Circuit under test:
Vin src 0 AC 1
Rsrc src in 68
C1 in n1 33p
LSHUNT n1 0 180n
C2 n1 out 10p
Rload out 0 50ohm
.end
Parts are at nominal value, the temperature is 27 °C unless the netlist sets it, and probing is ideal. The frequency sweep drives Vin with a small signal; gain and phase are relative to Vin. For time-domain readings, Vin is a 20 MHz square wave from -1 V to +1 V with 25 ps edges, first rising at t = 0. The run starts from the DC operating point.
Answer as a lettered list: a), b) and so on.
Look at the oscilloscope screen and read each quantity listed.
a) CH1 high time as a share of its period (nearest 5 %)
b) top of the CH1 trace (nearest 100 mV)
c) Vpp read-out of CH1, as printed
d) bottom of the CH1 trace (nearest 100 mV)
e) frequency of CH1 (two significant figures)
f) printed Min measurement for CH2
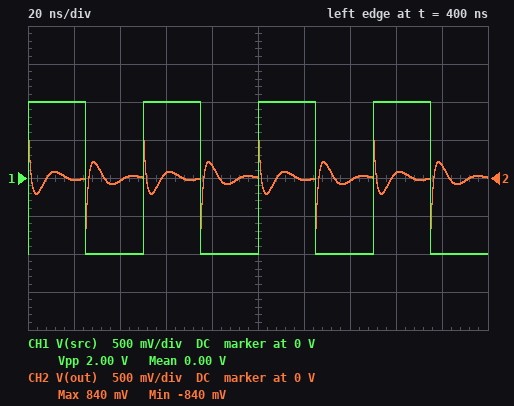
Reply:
a) 50 %
b) 1.0 V
c) 2.00 V
d) -1.0 V
e) 20 MHz
f) -840 mV
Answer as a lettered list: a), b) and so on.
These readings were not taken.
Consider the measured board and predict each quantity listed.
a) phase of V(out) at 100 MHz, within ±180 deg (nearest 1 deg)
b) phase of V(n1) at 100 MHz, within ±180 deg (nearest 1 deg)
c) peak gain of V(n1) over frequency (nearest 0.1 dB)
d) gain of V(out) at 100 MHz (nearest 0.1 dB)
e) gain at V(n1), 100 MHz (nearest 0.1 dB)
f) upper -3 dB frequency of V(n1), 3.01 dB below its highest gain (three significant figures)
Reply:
a) 90 deg
b) 17 deg
c) 2.0 dB
d) -10.6 dB
e) -0.1 dB
f) 115 MHz
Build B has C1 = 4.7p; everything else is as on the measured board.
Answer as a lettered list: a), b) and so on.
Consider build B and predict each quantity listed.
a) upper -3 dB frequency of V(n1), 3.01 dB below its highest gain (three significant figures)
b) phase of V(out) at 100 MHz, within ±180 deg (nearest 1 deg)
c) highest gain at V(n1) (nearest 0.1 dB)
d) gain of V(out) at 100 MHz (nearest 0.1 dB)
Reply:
a) 118 MHz
b) 158 deg
c) 1.7 dB
d) -8.8 dB
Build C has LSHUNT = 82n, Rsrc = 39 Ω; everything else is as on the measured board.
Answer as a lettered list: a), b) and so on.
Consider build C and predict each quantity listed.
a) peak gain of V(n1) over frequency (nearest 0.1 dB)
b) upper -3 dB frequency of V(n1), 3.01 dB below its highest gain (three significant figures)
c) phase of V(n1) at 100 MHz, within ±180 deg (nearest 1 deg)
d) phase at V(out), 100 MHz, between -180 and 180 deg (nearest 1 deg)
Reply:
a) 2.7 dB
b) 152 MHz
c) 57 deg
d) 129 deg
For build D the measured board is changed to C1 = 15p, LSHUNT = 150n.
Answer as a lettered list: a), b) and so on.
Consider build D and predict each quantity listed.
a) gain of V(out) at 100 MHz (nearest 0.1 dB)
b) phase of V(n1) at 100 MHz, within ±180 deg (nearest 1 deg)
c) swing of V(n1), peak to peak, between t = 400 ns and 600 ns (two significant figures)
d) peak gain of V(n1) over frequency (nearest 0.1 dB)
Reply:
a) -8.5 dB
b) 41 deg
c) 1.7 V
d) 3.2 dB
